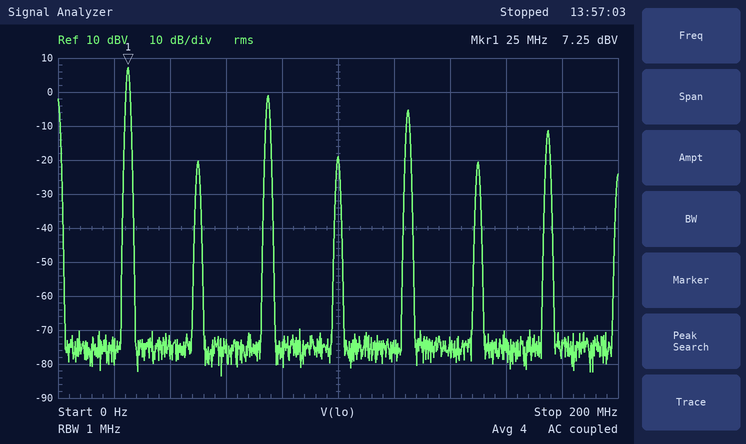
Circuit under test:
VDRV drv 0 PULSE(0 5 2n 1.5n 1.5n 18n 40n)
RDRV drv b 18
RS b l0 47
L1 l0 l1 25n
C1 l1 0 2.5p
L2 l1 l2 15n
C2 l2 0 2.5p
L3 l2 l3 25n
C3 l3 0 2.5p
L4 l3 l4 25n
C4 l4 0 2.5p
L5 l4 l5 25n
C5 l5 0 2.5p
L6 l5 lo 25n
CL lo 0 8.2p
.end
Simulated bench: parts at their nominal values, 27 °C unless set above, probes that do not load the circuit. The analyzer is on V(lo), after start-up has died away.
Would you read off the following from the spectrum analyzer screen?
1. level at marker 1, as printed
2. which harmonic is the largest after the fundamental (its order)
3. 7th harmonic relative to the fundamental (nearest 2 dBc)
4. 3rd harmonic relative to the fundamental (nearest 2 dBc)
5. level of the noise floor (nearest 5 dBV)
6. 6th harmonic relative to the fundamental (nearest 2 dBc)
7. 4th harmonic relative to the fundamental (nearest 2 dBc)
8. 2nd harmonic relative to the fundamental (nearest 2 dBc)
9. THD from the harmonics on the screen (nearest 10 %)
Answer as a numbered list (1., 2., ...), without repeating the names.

1. 7.25 dBV
2. 3
3. -18 dBc
4. -8 dBc
5. -75 dBV
6. -28 dBc
7. -26 dBc
8. -28 dBc
9. 50 %
